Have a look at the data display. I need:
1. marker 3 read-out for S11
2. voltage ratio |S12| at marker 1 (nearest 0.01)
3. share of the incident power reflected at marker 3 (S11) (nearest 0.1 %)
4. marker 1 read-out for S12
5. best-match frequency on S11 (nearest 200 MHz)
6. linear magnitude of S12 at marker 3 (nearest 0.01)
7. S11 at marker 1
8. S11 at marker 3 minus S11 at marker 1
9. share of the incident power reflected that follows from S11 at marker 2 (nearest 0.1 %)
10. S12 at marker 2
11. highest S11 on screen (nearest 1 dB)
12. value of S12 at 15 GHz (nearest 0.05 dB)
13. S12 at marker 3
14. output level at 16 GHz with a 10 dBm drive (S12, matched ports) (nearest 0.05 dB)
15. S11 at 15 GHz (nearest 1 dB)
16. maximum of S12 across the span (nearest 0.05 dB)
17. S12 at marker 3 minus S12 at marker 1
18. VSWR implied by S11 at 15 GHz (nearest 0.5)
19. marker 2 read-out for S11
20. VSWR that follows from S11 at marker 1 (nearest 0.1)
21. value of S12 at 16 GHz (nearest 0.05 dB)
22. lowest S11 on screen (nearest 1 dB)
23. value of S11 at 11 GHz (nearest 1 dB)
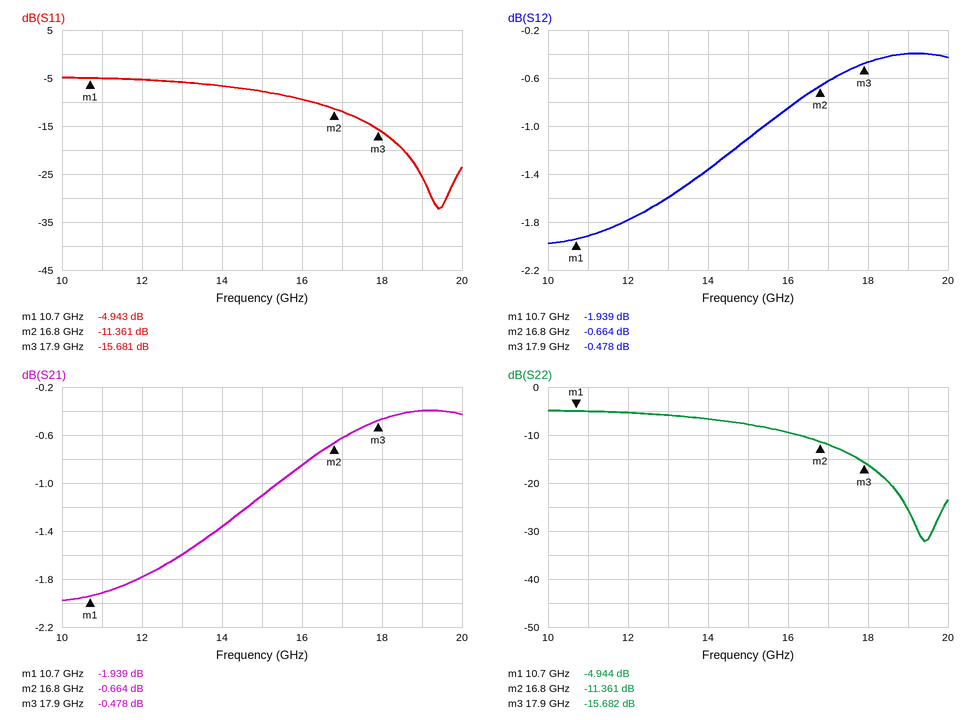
-15.681 dB
0.80
2.7 %
-1.939 dB
19.4 GHz
0.95
-4.943 dB
-10.738 dB
7.3 %
-0.664 dB
-5 dB
-1.10 dB
-0.478 dB
9.15 dBm
-8 dB
-0.40 dB
1.461 dB
2.5
-11.361 dB
3.6
-0.85 dB
-32 dB
-5 dB
